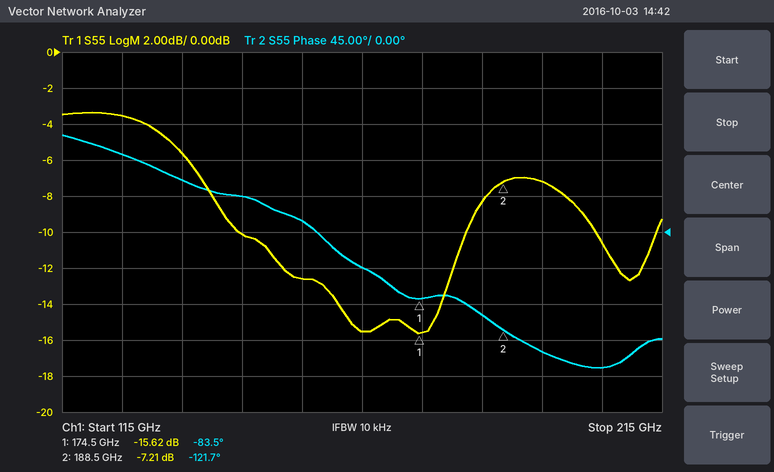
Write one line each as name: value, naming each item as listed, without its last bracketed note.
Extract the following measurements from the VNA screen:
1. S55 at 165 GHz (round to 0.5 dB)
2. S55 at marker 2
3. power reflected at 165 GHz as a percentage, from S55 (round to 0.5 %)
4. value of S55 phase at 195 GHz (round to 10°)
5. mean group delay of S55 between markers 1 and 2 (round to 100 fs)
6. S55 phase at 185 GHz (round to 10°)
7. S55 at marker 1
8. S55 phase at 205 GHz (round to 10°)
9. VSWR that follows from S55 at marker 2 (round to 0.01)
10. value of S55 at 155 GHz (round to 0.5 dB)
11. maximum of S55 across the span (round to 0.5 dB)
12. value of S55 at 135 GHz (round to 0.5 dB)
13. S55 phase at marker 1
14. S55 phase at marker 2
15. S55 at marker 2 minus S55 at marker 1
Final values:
S55 at 165 GHz: -15.5 dB
S55 at marker 2: -7.21 dB
power reflected at 165 GHz as a percentage, from S55: 3.0 %
value of S55 phase at 195 GHz: -150°
mean group delay of S55 between markers 1 and 2: 7.6 ps
S55 phase at 185 GHz: -100°
S55 at marker 1: -15.62 dB
S55 phase at 205 GHz: -170°
VSWR that follows from S55 at marker 2: 2.55
value of S55 at 155 GHz: -12.5 dB
maximum of S55 across the span: -3.5 dB
value of S55 at 135 GHz: -5.5 dB
S55 phase at marker 1: -83.5°
S55 phase at marker 2: -121.7°
S55 at marker 2 minus S55 at marker 1: 8.41 dB
